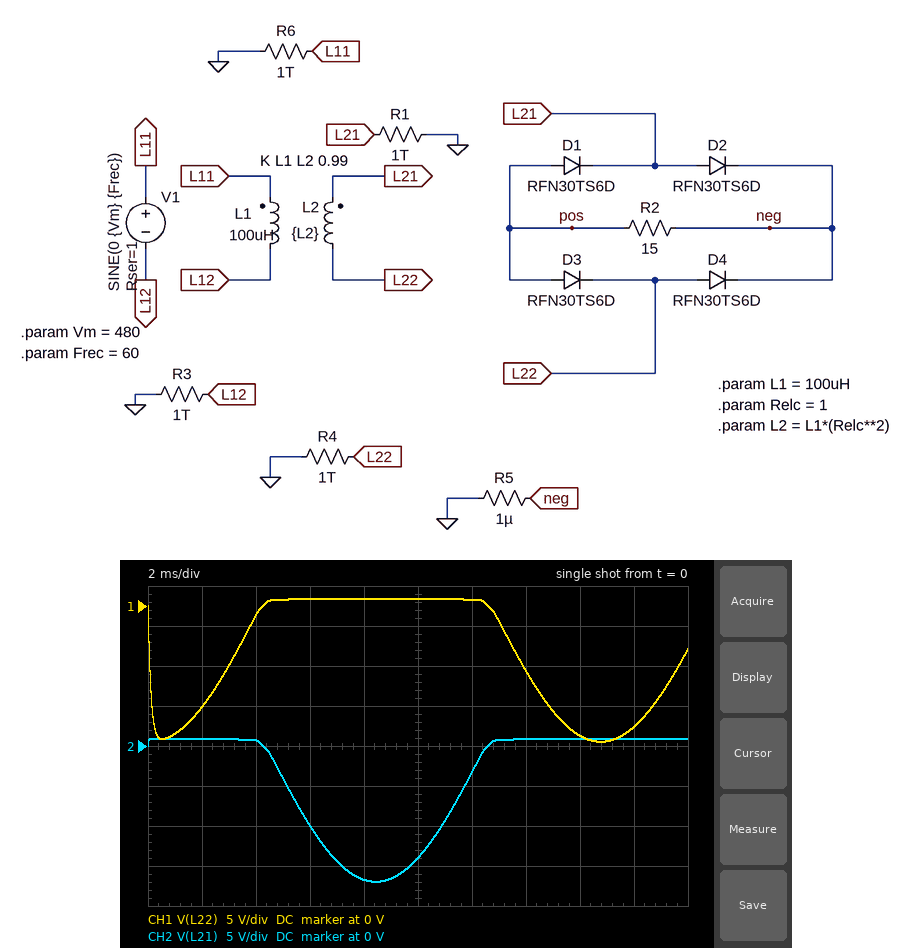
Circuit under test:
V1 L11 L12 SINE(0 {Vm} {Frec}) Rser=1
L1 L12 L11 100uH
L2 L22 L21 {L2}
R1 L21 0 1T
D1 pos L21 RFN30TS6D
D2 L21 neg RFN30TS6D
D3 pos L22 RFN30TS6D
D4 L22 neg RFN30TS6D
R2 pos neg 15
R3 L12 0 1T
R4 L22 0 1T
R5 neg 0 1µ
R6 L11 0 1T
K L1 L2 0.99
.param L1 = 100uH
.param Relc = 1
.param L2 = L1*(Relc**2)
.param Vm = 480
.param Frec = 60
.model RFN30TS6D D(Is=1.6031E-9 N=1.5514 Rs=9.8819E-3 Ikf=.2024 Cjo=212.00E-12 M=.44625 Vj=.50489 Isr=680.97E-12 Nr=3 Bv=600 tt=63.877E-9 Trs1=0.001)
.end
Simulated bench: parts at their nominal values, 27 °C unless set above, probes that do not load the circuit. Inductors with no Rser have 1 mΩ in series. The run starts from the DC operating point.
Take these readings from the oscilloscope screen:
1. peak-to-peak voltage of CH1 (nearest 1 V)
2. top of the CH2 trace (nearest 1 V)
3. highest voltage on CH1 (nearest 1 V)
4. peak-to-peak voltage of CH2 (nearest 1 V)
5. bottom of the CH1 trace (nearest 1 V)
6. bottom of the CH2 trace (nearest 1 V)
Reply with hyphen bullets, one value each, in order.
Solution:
- 18 V
- 1 V
- 1 V
- 18 V
- -17 V
- -17 V
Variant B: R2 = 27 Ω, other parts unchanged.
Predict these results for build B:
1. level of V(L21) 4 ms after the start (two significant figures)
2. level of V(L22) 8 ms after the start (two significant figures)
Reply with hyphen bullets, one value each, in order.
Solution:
- 660 mV
- 860 mV
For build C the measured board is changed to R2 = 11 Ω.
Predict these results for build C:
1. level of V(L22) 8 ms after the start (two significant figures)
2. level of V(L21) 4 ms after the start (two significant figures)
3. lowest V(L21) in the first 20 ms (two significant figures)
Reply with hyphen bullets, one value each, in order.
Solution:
- 930 mV
- 700 mV
- -17 V
